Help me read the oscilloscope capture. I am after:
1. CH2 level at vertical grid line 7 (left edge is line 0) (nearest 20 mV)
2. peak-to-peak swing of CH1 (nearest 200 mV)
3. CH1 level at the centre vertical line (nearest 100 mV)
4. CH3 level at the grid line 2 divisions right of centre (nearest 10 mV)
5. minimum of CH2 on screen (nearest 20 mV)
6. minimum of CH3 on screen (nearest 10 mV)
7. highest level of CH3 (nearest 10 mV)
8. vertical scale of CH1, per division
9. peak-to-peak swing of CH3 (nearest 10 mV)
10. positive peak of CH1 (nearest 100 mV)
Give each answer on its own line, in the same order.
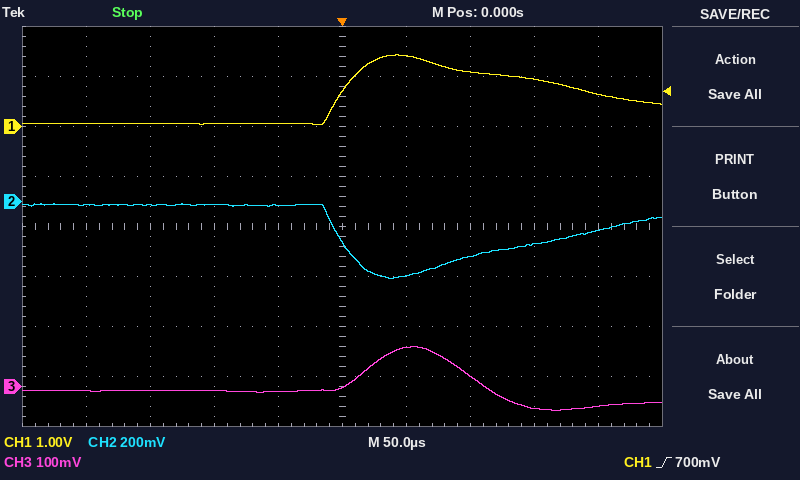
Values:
-220 mV
1.4 V
700 mV
20 mV
-300 mV
-50 mV
80 mV
1 V
130 mV
1.4 V
